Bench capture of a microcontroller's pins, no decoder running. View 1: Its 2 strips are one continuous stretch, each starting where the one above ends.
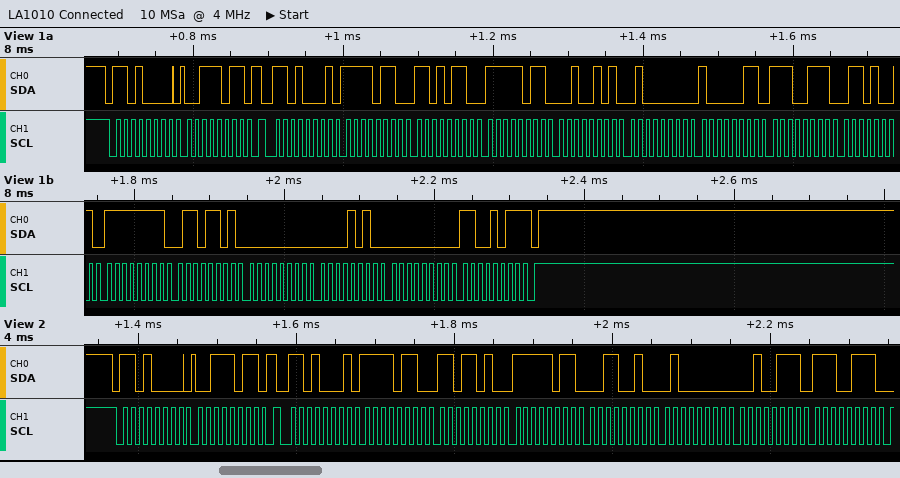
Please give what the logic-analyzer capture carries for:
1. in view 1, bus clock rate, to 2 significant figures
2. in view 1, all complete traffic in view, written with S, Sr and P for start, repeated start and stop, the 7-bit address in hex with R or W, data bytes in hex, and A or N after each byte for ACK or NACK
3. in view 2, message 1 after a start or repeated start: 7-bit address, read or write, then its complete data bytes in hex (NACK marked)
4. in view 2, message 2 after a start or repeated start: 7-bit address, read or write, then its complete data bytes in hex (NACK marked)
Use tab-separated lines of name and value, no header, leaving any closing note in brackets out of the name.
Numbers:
in view 1, bus clock rate, to 2 significant figures	100 kHz
in view 1, all complete traffic in view, written with S, Sr and P for start, repeated start and stop, the 7-bit address in hex with R or W, data bytes in hex, and A or N after each byte for ACK or NACK	S 68W A 3B A Sr 68R A F6 A D6 A FB A 25 A 40 A 83 A E7 A 69 A FF A 6D A 00 A 0A A 00 A CB N P
in view 2, message 1 after a start or repeated start: 7-bit address, read or write, then its complete data bytes in hex	0x68 write: 3B
in view 2, message 2 after a start or repeated start: 7-bit address, read or write, then its complete data bytes in hex	0x68 read: F6 DA FB 32 40 27 E7
